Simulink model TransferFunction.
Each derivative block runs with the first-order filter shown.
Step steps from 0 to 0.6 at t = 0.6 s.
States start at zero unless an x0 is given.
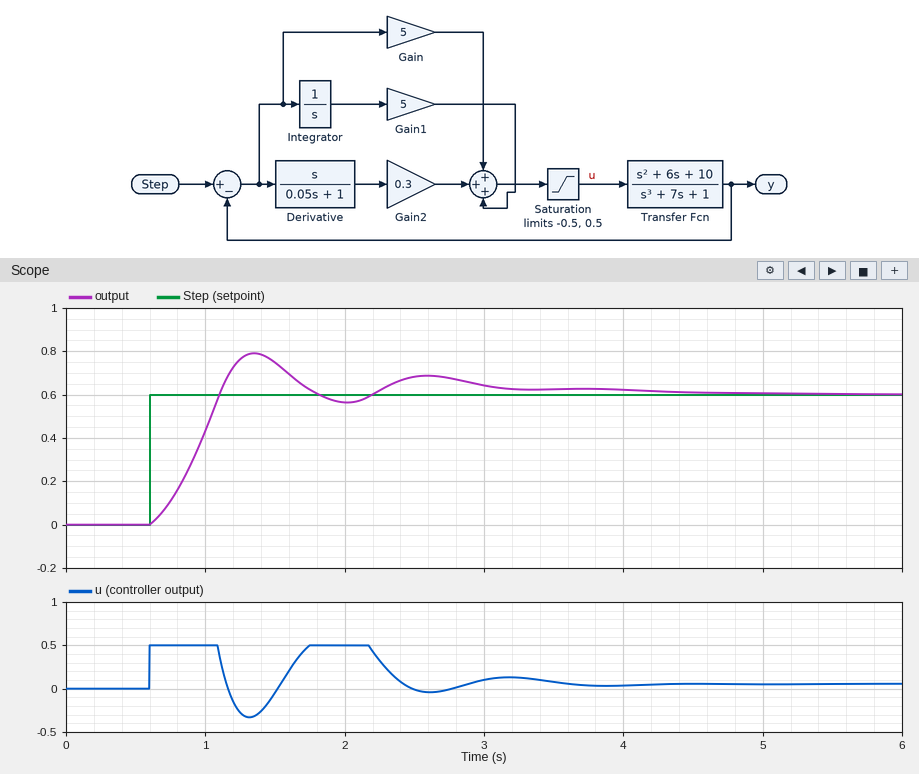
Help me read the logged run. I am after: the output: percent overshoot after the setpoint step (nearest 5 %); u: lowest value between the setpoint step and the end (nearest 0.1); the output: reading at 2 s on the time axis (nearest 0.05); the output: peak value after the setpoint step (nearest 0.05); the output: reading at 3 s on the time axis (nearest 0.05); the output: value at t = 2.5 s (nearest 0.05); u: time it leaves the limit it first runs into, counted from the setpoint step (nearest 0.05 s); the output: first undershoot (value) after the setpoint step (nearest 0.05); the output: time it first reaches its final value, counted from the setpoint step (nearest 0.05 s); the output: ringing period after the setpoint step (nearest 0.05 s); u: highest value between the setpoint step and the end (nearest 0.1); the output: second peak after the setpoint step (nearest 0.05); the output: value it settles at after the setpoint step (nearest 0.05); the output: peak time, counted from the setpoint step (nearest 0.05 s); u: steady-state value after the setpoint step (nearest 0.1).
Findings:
30 %
-0.3
0.55
0.80
0.65
0.70
0.50 s
0.55
0.50 s
1.25 s
0.5
0.70
0.60
0.75 s
0.1
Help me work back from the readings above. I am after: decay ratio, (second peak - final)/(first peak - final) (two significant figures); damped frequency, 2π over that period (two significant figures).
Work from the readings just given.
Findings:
0.50
5.0 rad/s
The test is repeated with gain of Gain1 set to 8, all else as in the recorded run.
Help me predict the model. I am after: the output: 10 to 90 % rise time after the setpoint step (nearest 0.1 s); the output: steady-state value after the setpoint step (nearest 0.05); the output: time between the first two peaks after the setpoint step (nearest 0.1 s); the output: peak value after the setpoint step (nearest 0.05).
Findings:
0.4 s
0.60
1.3 s
0.85
